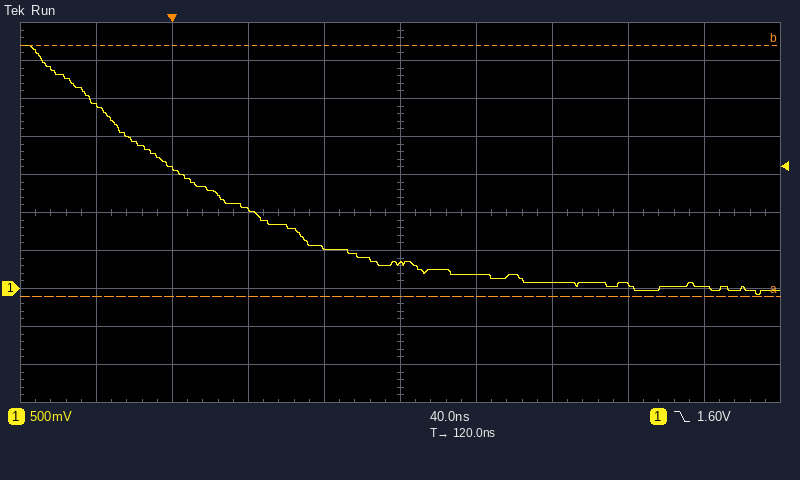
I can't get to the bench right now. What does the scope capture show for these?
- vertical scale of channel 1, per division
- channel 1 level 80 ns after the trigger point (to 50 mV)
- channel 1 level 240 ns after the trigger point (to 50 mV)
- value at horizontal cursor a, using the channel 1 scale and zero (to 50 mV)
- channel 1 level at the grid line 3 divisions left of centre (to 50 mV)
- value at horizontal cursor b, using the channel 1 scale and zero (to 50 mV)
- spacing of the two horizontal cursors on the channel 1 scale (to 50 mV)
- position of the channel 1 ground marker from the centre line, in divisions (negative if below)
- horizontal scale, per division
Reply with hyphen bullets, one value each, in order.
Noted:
- 500 mV
- 550 mV
- 50 mV
- -100 mV
- 1.60 V
- 3.20 V
- 3.30 V
- -2.0 div
- 40 ns
